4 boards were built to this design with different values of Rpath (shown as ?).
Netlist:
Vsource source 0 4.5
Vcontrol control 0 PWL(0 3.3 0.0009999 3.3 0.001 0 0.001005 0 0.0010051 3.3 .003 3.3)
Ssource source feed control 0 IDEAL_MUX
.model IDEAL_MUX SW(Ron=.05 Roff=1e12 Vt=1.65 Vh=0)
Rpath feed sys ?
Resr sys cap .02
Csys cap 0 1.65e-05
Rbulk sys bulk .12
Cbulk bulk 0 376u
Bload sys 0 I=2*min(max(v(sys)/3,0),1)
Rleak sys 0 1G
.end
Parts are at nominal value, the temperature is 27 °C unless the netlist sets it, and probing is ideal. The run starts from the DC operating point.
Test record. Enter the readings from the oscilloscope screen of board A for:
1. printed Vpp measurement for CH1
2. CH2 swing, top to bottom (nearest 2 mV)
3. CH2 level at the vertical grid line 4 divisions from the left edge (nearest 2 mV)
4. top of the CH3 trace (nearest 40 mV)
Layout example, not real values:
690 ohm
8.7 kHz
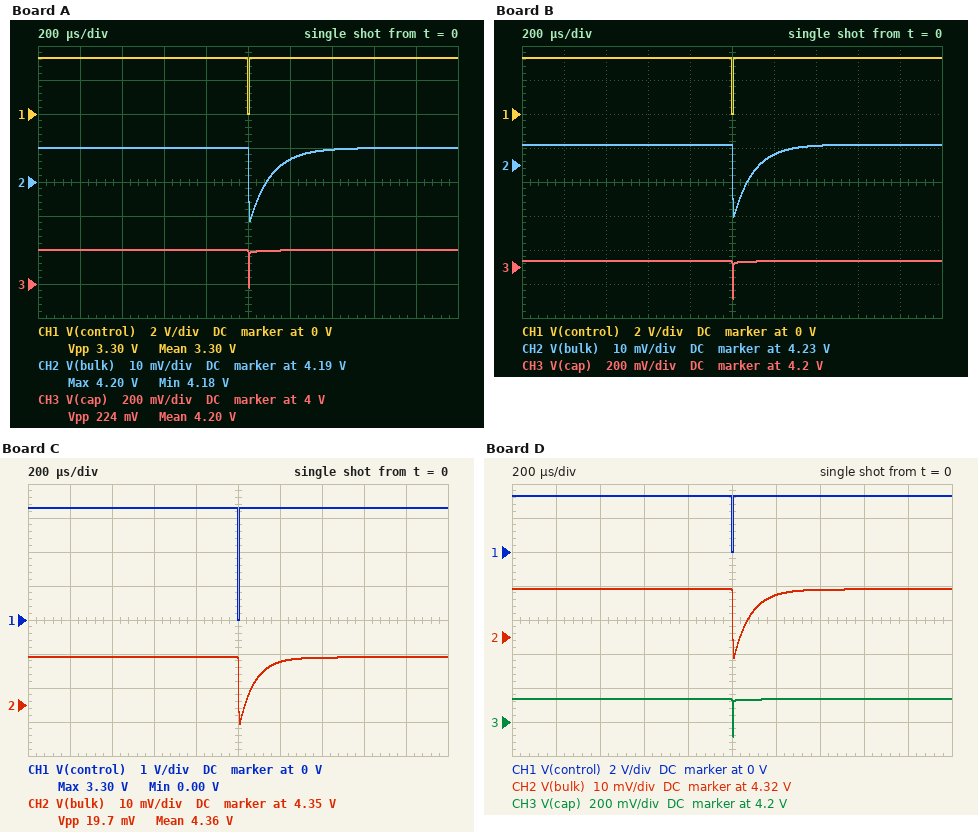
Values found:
3.30 V
22 mV
4.200 V
4.20 V
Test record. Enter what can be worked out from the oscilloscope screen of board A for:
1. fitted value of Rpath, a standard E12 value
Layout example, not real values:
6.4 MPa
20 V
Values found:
0.1 Ω
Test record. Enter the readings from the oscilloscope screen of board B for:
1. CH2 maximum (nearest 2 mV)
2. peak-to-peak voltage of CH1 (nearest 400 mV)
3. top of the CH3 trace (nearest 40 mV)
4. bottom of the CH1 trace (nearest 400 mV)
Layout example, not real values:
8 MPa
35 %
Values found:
4.236 V
3.2 V
4.24 V
0 V
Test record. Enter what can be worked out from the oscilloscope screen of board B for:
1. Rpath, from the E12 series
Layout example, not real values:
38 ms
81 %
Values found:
0.082 Ω
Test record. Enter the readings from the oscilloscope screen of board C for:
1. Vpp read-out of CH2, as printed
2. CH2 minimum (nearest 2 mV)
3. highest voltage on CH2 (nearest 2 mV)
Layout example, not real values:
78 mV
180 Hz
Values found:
19.7 mV
4.344 V
4.364 V
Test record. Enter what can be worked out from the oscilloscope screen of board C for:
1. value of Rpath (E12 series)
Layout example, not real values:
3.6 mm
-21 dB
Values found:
0.018 Ω
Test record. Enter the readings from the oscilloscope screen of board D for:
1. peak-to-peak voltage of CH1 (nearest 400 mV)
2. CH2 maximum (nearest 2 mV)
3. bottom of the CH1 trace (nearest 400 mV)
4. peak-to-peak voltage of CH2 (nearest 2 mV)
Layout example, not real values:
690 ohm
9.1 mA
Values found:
3.2 V
4.334 V
0 V
20 mV
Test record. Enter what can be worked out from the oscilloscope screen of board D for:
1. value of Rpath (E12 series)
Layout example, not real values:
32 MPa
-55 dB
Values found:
0.033 Ω
